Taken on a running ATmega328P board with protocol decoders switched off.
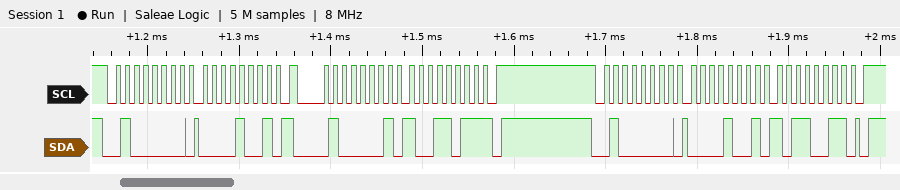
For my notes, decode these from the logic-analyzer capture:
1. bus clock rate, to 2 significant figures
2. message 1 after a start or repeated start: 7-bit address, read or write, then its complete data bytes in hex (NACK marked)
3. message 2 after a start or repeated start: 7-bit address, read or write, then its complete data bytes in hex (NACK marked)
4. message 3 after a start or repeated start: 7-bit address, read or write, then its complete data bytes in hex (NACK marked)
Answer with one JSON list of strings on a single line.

["100 kHz", "0x20 write: 09", "0x20 read: 9B NACK", "0x20 write: 09 B3"]
